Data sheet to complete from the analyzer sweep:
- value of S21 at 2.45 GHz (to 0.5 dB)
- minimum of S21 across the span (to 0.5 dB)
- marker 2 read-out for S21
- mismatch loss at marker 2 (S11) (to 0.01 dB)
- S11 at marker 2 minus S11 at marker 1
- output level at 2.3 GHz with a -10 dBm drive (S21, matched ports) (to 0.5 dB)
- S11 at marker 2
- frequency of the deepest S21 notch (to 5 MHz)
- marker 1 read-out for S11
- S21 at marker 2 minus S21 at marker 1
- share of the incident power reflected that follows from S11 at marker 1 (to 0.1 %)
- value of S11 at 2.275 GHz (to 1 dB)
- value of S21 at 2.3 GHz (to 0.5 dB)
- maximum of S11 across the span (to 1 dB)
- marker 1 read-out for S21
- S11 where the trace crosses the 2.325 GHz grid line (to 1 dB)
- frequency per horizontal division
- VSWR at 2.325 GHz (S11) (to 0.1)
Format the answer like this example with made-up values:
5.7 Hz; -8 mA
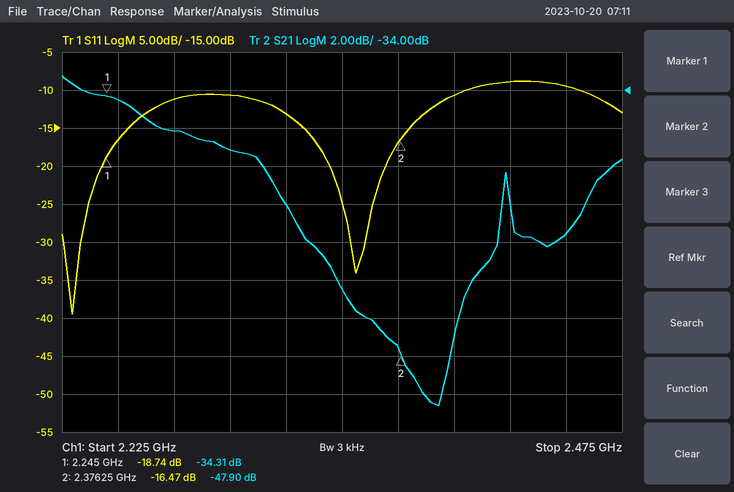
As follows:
-41.5 dB; -50.5 dB; -47.90 dB; 0.10 dB; 2.27 dB; -47.0 dBm; -16.47 dB; 2.395 GHz; -18.74 dB; -13.59 dB; 1.3 %; -11 dB; -37.0 dB; -9 dB; -34.31 dB; -13 dB; 25 MHz; 1.6
